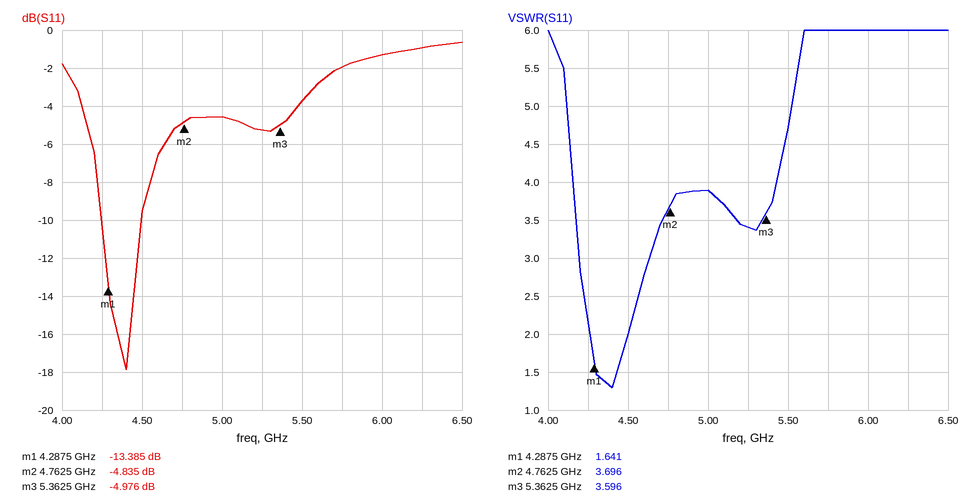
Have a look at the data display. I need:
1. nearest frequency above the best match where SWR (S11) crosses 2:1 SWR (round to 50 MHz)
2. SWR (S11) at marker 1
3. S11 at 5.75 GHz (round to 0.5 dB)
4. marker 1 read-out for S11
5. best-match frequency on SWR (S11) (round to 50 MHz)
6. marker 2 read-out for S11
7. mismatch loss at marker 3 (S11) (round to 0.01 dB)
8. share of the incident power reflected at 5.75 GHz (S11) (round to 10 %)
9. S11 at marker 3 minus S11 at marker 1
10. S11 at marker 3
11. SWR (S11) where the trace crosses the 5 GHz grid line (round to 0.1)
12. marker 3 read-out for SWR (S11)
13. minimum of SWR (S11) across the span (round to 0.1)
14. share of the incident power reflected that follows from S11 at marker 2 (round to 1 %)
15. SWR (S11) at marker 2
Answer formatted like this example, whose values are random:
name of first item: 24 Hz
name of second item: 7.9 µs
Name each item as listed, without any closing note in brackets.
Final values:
nearest frequency above the best match where SWR (S11) crosses 2:1 SWR: 4.50 GHz
SWR (S11) at marker 1: 1.641
S11 at 5.75 GHz: -2.0 dB
marker 1 read-out for S11: -13.385 dB
best-match frequency on SWR (S11): 4.40 GHz
marker 2 read-out for S11: -4.835 dB
mismatch loss at marker 3 (S11): 1.66 dB
share of the incident power reflected at 5.75 GHz (S11): 60 %
S11 at marker 3 minus S11 at marker 1: 8.409 dB
S11 at marker 3: -4.976 dB
SWR (S11) where the trace crosses the 5 GHz grid line: 3.9
marker 3 read-out for SWR: 3.596
minimum of SWR (S11) across the span: 1.3
share of the incident power reflected that follows from S11 at marker 2: 33 %
SWR (S11) at marker 2: 3.696
